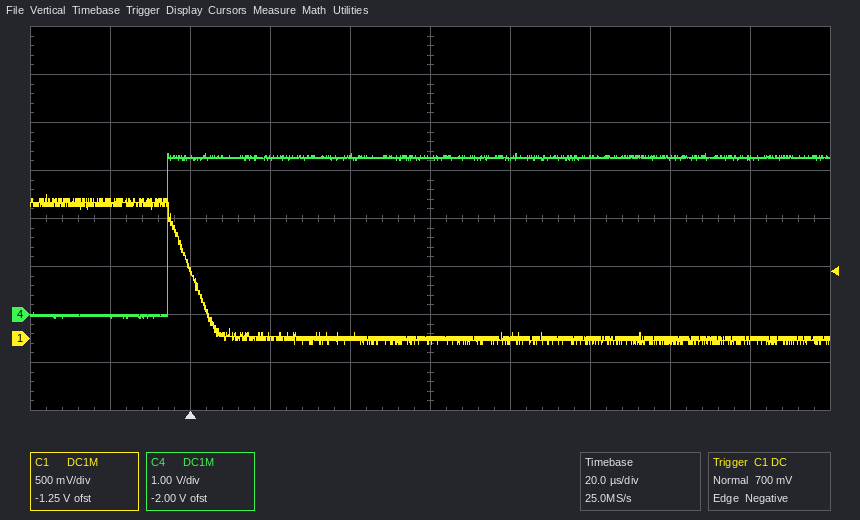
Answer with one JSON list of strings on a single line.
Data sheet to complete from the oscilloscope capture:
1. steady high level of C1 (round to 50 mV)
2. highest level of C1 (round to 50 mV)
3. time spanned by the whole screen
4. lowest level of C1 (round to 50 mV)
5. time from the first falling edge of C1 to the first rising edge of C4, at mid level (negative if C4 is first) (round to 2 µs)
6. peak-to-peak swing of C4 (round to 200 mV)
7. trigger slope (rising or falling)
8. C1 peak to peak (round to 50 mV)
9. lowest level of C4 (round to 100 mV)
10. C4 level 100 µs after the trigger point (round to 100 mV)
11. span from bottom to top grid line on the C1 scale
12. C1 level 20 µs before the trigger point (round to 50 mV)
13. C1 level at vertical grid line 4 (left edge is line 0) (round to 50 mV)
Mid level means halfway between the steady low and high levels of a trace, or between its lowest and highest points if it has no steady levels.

["1.40 V", "1.50 V", "200 µs", "-50 mV", "-6 µs", "3.4 V", "falling", "1.55 V", "-100 mV", "3.3 V", "4 V", "1.40 V", "0 mV"]
